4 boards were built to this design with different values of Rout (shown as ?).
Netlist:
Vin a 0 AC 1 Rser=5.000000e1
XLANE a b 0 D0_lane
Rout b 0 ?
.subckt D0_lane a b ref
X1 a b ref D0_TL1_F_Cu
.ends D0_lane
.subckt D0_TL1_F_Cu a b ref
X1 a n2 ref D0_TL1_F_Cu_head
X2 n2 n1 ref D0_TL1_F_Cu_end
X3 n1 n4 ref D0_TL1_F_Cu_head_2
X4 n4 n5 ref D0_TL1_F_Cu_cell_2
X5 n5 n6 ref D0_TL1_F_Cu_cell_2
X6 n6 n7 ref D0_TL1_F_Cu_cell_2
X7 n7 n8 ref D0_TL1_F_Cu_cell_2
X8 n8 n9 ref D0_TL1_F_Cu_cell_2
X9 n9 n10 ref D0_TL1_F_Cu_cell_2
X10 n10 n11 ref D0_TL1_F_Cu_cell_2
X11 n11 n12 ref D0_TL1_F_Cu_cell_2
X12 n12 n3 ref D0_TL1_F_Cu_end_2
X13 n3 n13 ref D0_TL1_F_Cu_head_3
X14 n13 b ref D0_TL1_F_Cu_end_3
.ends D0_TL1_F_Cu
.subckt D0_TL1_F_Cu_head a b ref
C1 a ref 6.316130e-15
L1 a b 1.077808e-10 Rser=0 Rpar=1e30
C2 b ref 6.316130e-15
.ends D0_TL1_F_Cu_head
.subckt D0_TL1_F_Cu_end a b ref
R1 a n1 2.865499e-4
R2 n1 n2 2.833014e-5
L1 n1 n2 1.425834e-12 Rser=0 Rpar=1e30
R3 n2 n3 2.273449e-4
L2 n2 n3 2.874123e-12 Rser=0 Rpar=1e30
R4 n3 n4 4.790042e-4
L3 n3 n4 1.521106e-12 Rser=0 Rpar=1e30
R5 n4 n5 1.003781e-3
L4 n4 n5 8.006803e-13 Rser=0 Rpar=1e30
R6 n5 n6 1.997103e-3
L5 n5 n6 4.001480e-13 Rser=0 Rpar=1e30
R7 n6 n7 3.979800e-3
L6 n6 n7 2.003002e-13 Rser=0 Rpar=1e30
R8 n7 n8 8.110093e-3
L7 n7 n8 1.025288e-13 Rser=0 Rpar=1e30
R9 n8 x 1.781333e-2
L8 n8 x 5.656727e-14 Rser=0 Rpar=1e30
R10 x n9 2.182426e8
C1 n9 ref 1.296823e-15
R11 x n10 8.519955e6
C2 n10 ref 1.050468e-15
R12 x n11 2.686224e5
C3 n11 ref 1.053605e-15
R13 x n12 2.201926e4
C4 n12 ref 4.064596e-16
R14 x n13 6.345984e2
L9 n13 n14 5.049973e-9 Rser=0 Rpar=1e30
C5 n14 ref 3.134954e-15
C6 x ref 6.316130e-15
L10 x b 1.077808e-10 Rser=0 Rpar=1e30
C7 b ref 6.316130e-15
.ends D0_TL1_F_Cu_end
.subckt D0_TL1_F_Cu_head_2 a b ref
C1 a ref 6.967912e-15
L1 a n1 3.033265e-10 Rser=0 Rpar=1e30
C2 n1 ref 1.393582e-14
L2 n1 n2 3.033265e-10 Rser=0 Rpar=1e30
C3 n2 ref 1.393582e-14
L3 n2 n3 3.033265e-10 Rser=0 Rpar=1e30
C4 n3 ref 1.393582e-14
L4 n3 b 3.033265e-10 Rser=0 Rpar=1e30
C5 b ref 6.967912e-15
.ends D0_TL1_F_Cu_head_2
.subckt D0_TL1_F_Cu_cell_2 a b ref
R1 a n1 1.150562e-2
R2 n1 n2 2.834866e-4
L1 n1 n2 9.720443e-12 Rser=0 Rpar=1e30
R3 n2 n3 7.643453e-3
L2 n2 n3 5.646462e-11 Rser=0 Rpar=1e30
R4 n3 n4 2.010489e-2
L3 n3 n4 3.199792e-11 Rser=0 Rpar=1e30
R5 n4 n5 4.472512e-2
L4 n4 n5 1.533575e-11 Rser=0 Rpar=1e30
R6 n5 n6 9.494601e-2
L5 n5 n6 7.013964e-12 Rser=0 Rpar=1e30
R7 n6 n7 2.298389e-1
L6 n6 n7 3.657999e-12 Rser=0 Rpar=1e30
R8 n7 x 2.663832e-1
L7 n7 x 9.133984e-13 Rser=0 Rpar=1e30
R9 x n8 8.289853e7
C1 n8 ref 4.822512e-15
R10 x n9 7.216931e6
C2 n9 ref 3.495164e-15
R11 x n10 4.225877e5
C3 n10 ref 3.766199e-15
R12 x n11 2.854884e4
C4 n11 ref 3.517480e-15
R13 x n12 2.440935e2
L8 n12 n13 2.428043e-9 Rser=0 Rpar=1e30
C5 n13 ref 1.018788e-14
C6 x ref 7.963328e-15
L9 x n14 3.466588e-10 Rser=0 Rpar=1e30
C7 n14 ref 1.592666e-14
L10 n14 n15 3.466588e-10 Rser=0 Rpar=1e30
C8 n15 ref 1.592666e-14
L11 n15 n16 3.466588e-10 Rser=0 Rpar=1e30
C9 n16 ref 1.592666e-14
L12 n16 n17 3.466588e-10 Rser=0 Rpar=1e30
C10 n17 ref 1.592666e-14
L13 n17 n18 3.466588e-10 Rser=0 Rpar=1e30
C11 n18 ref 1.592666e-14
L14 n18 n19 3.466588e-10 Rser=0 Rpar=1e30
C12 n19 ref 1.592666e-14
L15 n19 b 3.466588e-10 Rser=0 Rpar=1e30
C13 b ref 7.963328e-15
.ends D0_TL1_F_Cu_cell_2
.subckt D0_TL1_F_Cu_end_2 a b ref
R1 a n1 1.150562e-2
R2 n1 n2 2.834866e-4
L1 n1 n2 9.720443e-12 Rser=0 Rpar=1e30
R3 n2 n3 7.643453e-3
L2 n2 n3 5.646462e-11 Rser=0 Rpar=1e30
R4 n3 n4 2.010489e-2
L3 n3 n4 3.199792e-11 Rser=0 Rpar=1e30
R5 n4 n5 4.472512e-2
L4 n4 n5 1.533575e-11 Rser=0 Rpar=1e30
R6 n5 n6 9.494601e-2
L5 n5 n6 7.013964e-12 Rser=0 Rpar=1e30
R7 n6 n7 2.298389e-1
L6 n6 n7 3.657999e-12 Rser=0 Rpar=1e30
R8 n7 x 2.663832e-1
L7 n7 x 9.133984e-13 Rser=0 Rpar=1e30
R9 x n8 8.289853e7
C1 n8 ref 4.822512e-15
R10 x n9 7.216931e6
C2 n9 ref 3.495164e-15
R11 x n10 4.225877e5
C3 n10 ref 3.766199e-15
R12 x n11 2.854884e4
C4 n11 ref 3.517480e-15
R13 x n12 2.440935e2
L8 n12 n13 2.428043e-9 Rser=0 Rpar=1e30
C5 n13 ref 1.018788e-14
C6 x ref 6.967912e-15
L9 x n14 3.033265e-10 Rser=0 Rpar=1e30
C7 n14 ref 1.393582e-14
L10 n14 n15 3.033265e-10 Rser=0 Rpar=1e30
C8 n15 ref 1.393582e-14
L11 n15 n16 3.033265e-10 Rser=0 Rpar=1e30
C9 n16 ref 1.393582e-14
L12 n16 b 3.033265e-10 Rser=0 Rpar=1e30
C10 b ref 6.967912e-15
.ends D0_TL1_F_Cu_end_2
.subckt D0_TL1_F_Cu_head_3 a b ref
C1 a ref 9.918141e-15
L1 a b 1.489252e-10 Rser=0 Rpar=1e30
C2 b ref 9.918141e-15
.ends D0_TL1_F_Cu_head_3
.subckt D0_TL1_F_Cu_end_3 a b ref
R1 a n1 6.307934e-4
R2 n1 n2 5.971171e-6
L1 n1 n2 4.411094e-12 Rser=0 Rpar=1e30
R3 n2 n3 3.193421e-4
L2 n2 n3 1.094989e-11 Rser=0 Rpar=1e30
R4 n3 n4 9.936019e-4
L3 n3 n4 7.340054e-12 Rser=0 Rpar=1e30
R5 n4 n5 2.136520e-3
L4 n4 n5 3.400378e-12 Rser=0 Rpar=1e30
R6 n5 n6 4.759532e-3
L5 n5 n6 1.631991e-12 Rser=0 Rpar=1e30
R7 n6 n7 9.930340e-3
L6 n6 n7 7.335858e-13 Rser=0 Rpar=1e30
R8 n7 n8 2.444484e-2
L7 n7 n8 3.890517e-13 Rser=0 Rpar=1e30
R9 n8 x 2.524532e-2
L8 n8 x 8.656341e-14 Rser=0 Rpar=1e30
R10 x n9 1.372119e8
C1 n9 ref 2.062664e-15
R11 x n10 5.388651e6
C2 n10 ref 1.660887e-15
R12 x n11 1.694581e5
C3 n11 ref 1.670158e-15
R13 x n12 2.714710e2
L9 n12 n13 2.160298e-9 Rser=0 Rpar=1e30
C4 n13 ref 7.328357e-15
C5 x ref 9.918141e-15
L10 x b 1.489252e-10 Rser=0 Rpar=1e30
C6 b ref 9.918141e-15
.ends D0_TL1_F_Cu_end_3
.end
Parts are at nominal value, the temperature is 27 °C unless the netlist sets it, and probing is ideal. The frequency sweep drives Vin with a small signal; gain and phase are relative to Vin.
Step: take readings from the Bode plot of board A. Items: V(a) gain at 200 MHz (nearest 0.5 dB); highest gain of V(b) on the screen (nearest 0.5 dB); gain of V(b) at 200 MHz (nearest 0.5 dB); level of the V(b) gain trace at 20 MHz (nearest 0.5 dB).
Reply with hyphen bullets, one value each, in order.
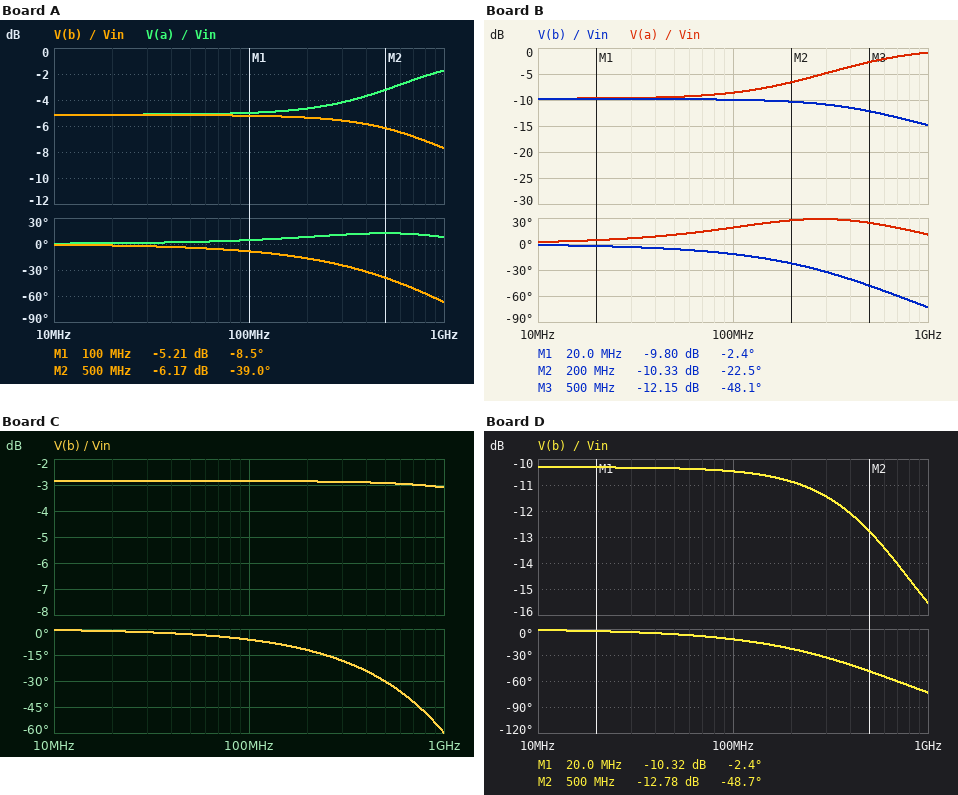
- -4.5 dB
- -5.0 dB
- -5.5 dB
- -5.0 dB
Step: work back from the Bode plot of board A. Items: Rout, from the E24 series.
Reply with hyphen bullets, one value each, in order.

- 62 Ω
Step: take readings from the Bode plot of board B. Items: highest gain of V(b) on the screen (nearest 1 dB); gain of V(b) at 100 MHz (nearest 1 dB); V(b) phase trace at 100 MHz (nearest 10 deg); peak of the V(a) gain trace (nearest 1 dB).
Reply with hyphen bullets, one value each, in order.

- -10 dB
- -10 dB
- -10 deg
- -1 dB
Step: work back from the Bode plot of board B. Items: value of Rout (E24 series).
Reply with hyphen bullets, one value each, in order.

- 24 Ω
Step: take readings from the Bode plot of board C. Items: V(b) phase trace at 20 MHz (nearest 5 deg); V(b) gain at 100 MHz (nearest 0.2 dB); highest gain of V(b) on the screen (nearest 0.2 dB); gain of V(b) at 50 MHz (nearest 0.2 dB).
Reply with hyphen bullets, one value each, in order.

- 0 deg
- -2.8 dB
- -2.8 dB
- -2.8 dB
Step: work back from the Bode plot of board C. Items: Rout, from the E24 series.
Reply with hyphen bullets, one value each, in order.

- 130 Ω
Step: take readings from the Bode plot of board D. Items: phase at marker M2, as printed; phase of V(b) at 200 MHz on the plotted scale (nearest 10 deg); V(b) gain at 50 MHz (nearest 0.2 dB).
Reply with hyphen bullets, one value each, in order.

- -48.7 deg
- -20 deg
- -10.4 dB
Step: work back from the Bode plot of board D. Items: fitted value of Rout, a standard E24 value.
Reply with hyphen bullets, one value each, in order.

- 22 Ω
